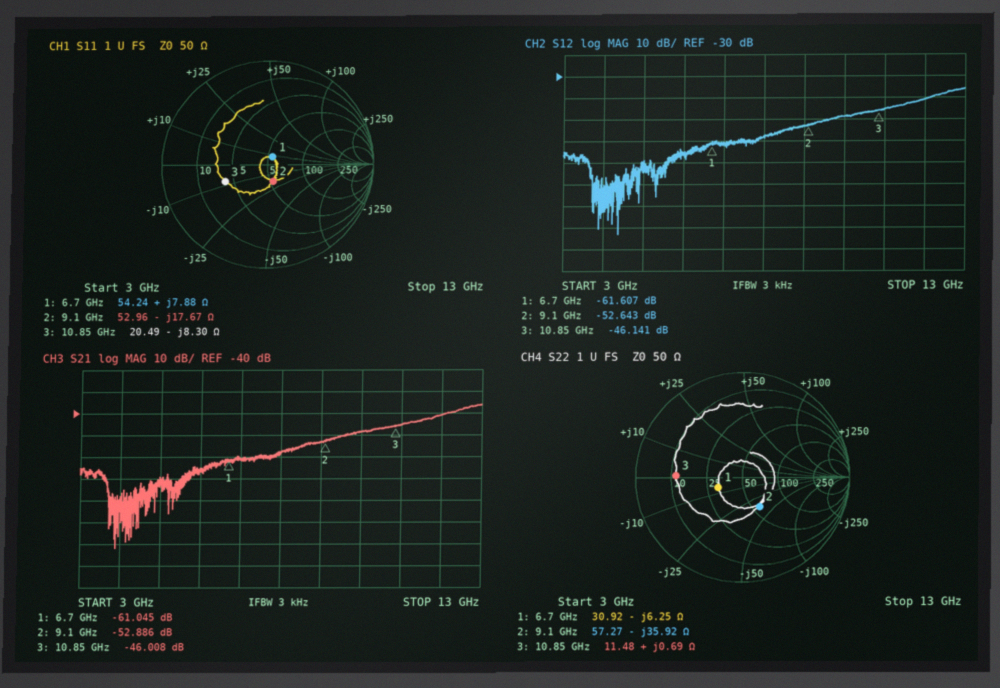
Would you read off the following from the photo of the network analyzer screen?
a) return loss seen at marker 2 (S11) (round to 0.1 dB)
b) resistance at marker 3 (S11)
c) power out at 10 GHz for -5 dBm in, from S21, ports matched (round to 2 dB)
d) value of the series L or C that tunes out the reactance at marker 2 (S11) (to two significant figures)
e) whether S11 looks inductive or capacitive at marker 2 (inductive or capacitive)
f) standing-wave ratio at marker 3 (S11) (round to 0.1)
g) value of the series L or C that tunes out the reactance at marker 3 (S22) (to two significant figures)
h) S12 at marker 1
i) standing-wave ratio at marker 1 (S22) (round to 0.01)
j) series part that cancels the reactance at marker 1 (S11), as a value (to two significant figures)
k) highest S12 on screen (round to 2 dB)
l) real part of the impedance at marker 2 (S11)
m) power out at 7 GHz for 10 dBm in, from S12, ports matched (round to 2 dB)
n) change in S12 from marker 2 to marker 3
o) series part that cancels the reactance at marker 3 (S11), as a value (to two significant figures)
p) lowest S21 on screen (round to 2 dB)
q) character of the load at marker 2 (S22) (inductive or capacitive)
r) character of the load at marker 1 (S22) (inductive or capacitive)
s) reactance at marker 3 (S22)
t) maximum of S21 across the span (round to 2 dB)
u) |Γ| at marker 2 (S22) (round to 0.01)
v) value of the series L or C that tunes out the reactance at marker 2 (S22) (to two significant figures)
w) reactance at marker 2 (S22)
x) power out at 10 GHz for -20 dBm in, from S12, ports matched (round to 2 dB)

15.3 dB
20.49 Ω
-54 dBm
310 pH
capacitive
2.5
21 pF
-61.607 dB
1.66
3.0 pF
-36 dB
52.96 Ω
-52 dBm
6.502 dB
120 pH
-102 dB
capacitive
capacitive
+0.69 Ω
-36 dB
0.32
630 pH
-35.92 Ω
-68 dBm
